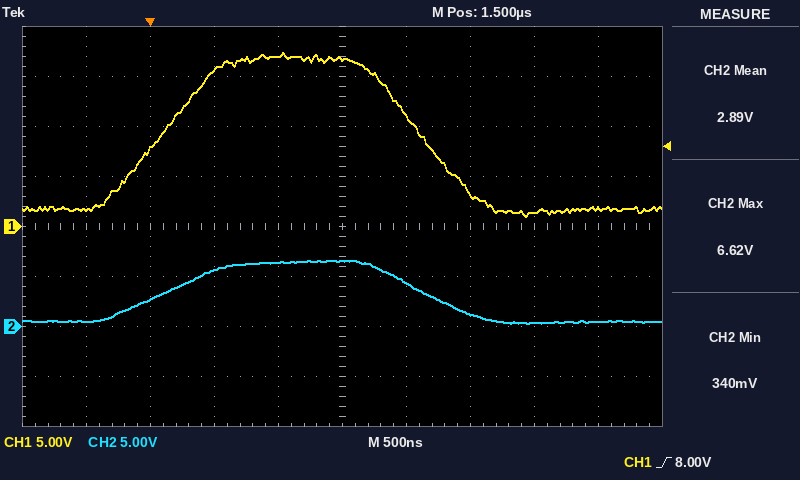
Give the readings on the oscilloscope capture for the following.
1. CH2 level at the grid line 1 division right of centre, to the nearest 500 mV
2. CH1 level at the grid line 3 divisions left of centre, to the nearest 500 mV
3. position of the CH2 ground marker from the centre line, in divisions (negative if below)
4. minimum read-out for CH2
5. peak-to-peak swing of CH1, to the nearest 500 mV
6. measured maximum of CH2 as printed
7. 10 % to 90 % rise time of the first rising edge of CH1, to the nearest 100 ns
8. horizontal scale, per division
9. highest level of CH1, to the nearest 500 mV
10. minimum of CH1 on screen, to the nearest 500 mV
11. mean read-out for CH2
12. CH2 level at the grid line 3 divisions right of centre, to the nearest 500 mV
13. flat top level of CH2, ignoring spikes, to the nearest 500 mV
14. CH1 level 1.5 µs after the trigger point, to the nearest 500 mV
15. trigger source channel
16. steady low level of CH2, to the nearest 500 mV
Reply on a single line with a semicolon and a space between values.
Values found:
4.5 V; 7.5 V; -2.0 div; 340 mV; 16.5 V; 6.62 V; 800 ns; 500 ns; 17.5 V; 1.0 V; 2.89 V; 500 mV; 6.5 V; 17.0 V; CH1; 500 mV
